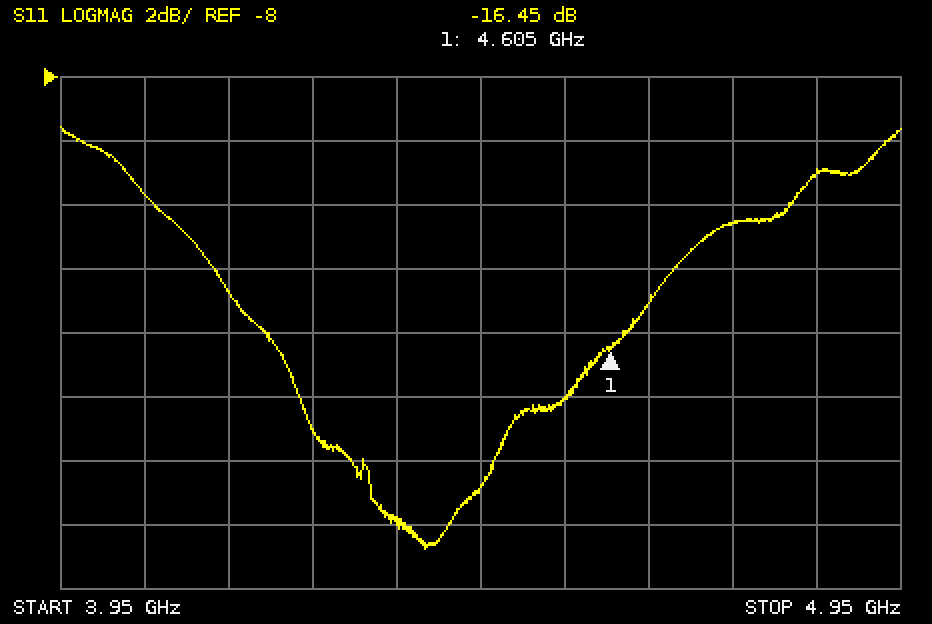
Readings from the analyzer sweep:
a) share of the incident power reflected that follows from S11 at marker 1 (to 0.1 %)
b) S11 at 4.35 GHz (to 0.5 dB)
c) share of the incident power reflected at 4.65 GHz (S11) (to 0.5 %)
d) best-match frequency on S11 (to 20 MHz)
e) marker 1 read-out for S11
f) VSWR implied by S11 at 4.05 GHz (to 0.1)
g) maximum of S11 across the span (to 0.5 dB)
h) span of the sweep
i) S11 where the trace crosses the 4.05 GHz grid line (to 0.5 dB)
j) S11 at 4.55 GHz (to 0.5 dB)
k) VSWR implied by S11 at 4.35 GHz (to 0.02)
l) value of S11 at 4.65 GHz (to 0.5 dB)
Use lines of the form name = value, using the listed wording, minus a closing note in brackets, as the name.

share of the incident power reflected that follows from S11 at marker 1 = 2.3 %
S11 at 4.35 GHz = -22.0 dB
share of the incident power reflected at 4.65 GHz (S11) = 3.0 %
best-match frequency on S11 = 4.38 GHz
marker 1 read-out for S11 = -16.45 dB
VSWR implied by S11 at 4.05 GHz = 1.7
maximum of S11 across the span = -9.5 dB
span of the sweep = 1 GHz
S11 where the trace crosses the 4.05 GHz grid line = -11.5 dB
S11 at 4.55 GHz = -18.0 dB
VSWR implied by S11 at 4.35 GHz = 1.18
value of S11 at 4.65 GHz = -15.0 dB
